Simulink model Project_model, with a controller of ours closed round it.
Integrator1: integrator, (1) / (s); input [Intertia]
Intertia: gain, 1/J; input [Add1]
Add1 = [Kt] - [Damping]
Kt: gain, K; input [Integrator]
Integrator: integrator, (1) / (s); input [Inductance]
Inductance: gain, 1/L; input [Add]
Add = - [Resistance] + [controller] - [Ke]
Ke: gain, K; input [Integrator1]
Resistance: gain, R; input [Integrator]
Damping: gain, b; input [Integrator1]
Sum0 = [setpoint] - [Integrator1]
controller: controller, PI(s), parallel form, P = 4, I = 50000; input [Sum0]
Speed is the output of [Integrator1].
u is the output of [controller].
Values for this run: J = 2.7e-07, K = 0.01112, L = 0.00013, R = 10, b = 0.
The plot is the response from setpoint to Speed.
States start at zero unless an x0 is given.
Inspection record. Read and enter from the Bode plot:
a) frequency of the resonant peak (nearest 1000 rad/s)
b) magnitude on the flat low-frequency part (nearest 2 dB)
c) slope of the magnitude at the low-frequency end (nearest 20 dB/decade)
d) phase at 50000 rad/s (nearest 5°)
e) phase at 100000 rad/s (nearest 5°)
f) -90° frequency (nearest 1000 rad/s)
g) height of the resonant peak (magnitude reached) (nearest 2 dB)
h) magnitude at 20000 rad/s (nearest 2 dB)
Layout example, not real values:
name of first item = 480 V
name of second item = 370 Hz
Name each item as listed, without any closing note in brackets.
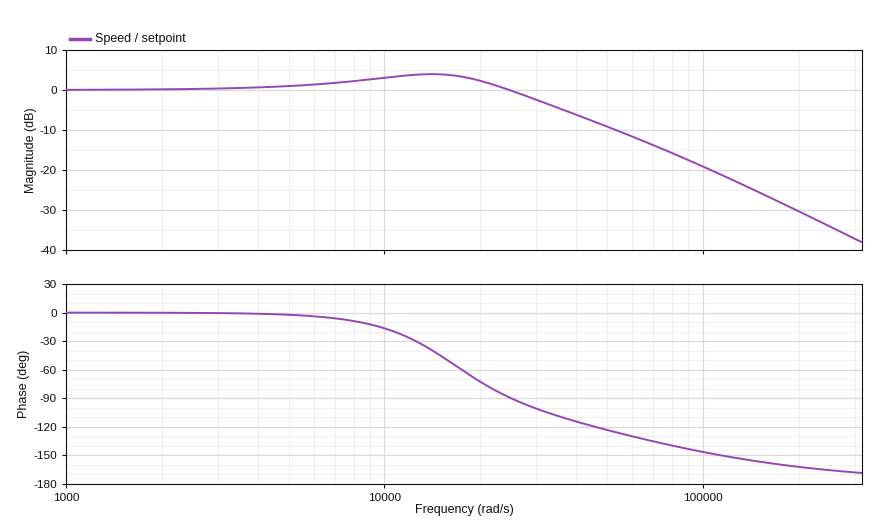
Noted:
frequency of the resonant peak = 14000 rad/s
magnitude on the flat low-frequency part = 0 dB
slope of the magnitude at the low-frequency end = 0 dB/decade
phase at 50000 rad/s = -125°
phase at 100000 rad/s = -145°
-90° frequency = 25000 rad/s
height of the resonant peak (magnitude reached) = 4 dB
magnitude at 20000 rad/s = 2 dB
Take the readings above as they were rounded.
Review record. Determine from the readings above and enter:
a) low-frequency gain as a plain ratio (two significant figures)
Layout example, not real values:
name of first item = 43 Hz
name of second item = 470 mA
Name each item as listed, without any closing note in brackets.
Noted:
low-frequency gain as a plain ratio = 1.0
